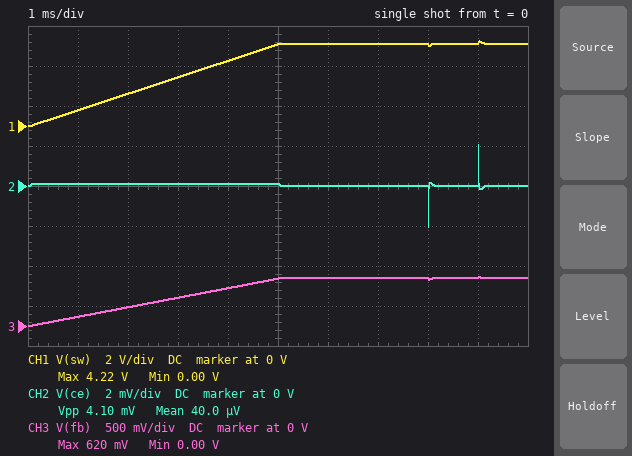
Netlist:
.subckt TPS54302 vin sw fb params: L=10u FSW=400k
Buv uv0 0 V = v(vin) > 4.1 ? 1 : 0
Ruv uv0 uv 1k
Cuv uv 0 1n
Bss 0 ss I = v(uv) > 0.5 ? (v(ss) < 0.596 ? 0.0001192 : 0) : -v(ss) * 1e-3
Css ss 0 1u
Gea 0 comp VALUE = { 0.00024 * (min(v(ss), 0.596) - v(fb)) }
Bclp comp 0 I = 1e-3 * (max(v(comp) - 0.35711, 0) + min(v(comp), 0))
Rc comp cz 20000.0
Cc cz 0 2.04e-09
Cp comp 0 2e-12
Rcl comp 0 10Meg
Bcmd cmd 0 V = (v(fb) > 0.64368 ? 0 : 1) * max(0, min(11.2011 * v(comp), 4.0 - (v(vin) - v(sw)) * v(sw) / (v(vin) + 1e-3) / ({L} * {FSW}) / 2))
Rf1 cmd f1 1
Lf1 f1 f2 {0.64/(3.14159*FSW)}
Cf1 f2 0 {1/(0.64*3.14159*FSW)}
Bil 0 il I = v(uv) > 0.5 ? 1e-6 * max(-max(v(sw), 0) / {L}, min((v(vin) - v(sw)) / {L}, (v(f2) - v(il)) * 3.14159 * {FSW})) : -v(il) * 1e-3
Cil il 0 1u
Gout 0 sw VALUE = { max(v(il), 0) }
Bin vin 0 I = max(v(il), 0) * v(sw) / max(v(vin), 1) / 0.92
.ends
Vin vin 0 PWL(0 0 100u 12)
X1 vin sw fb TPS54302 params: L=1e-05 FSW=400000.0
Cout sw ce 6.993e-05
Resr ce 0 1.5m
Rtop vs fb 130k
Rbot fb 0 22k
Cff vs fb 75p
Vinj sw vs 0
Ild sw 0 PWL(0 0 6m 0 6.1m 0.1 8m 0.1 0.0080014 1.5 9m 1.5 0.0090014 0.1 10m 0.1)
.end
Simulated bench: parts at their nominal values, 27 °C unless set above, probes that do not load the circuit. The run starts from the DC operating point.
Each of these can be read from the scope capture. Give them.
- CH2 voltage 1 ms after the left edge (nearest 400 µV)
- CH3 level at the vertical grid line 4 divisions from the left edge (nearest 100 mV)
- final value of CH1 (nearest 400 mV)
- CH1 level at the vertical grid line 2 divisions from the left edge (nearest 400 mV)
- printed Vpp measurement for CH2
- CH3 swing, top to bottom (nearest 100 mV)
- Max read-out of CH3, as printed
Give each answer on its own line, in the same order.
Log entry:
0 V
500 mV
4.0 V
1.6 V
4.10 mV
600 mV
620 mV
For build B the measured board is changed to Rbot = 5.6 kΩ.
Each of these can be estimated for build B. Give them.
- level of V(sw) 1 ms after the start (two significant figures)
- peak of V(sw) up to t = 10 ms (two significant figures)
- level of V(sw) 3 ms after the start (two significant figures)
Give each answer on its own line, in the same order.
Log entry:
2.8 V
13 V
8.5 V
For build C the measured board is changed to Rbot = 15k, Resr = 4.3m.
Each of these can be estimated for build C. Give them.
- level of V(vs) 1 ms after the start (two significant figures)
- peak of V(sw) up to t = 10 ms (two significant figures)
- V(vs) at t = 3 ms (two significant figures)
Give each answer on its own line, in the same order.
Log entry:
1.1 V
5.9 V
3.4 V
